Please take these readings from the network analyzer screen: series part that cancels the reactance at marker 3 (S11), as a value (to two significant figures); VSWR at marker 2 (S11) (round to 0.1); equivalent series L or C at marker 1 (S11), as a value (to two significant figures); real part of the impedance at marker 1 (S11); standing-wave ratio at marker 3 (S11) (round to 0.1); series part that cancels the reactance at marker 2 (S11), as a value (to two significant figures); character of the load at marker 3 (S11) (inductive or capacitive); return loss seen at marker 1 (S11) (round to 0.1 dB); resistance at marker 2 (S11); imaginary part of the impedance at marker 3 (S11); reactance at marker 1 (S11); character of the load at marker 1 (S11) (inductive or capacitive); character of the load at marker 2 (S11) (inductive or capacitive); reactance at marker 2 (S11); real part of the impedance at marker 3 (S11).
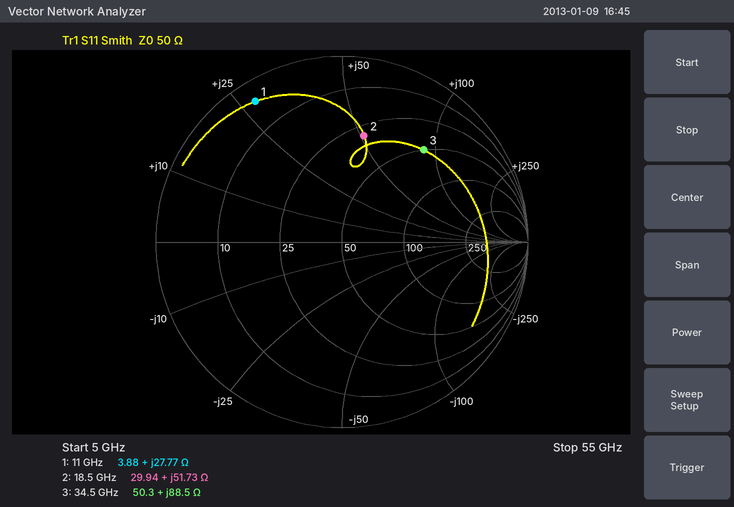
52 fF
3.8
400 pH
3.88 Ω
4.9
170 fF
inductive
1.0 dB
29.94 Ω
+88.5 Ω
+27.77 Ω
inductive
inductive
+51.73 Ω
50.3 Ω
